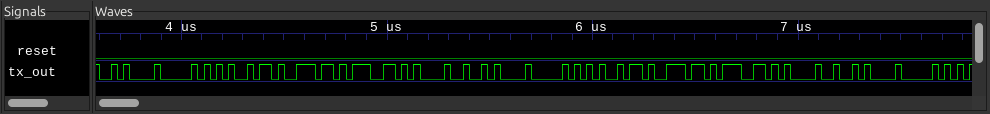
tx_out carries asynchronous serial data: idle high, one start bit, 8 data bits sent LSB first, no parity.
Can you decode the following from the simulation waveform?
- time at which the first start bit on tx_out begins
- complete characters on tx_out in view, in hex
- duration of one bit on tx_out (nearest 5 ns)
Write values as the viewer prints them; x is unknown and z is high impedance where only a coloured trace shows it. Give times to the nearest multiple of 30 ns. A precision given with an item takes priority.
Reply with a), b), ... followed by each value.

a) 3600 ns
b) 0A, 50, 69, 6E, 67, 21, 0A, 50, 69, 6E, 67, 21, 0A, 50
c) 30 ns
